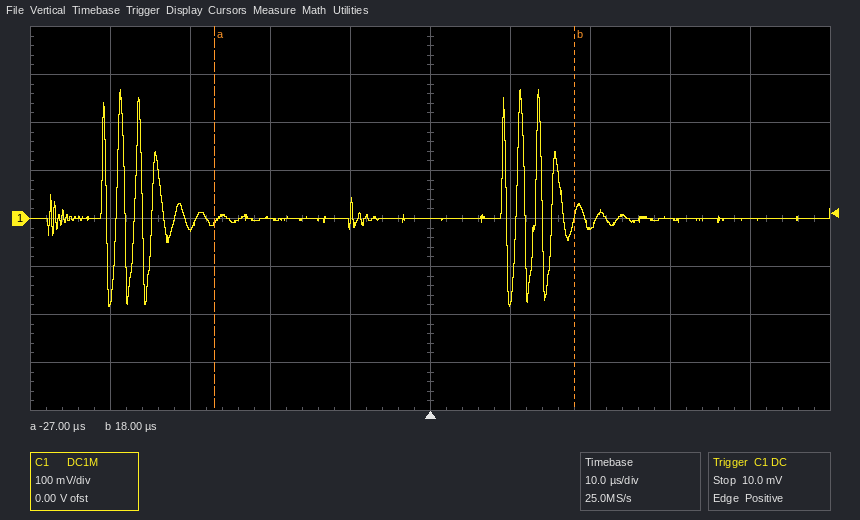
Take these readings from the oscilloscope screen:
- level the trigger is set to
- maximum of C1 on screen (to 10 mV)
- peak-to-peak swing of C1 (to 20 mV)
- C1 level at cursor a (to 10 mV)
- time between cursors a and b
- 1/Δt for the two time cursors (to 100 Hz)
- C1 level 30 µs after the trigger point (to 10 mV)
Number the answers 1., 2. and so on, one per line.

1. 10.0 mV
2. 270 mV
3. 460 mV
4. -10 mV
5. 45 µs
6. 22.2 kHz
7. 0 mV
